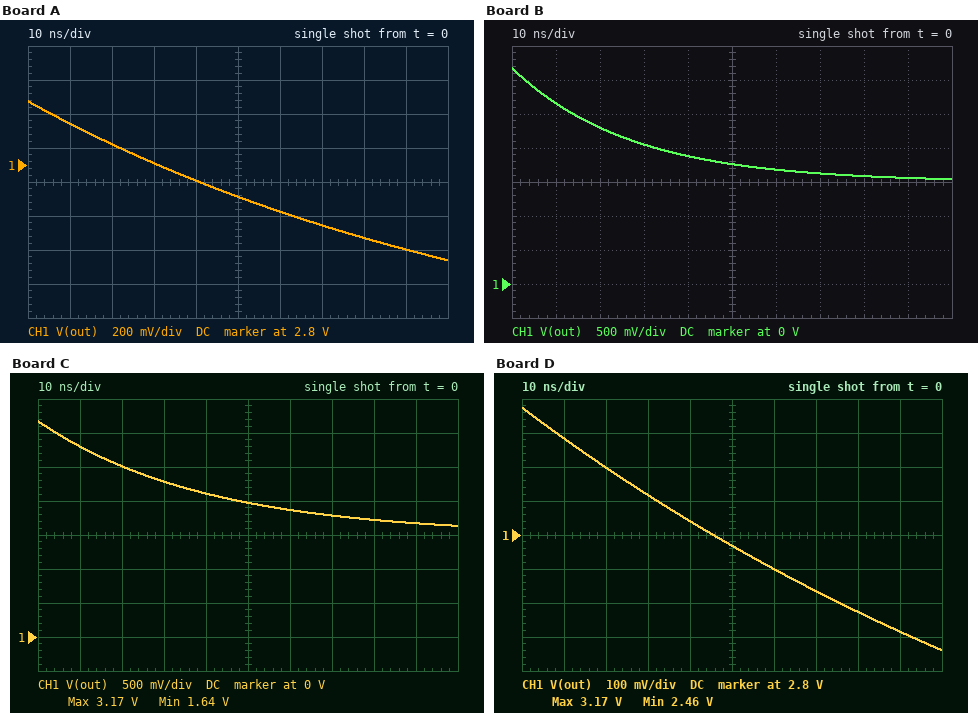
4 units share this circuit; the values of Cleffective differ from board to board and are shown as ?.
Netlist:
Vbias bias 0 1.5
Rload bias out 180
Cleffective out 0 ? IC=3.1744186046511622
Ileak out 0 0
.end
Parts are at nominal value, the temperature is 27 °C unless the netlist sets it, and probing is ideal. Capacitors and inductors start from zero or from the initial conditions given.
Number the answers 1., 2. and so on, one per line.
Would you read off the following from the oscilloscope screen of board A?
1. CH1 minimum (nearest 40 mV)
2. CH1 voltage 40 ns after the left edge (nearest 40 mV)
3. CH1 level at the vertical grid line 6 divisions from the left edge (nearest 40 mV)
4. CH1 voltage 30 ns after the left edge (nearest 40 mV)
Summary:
1. 2.24 V
2. 2.72 V
3. 2.52 V
4. 2.80 V
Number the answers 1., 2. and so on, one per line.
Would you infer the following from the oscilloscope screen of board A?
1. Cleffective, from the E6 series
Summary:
1. 680 pF
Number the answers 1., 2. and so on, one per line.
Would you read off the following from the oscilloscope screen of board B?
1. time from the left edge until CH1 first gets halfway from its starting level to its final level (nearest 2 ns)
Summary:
1. 18 ns
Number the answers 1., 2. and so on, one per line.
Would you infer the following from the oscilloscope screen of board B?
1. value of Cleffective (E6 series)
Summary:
1. 150 pF
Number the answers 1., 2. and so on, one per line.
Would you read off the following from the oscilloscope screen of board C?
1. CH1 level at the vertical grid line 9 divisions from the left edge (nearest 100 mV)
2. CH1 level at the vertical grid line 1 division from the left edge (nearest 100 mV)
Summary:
1. 1.7 V
2. 2.8 V
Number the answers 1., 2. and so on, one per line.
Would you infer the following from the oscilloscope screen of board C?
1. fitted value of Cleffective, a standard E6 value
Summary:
1. 220 pF
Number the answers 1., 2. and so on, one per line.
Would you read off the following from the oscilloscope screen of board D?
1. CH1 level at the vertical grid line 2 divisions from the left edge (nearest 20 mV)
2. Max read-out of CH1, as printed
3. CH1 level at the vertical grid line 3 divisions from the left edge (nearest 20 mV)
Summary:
1. 3.00 V
2. 3.17 V
3. 2.92 V
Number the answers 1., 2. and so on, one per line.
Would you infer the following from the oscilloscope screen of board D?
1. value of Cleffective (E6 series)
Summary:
1. 1 nF
